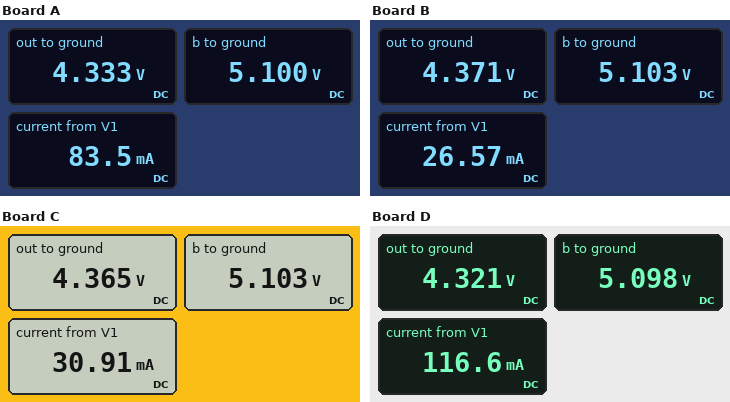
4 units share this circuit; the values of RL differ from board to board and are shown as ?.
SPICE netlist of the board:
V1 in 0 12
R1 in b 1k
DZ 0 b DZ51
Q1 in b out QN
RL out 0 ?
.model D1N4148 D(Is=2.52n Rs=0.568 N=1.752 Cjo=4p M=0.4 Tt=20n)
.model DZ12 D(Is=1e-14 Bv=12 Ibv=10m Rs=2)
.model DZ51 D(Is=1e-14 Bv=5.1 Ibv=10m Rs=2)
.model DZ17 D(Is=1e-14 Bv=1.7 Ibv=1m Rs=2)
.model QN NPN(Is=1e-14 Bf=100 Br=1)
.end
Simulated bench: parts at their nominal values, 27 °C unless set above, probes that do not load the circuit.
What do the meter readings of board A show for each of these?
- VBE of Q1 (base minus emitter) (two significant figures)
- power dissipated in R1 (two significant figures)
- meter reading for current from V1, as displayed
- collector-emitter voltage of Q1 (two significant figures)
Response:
770 mV
48 mW
83.5 mA
7.7 V
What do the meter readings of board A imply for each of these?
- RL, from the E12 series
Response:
56 Ω
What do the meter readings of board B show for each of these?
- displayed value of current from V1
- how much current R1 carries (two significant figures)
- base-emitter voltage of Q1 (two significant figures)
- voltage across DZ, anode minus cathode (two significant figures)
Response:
26.57 mA
6.9 mA
730 mV
-5.1 V
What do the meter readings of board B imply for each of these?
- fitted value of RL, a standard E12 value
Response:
220 Ω
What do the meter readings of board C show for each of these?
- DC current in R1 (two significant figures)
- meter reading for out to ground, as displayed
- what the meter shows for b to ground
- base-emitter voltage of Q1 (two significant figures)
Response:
6.9 mA
4.365 V
5.103 V
740 mV
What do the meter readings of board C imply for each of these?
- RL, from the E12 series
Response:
180 Ω
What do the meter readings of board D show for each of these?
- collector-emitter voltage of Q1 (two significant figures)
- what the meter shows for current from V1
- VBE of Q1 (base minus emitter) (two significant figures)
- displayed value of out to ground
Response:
7.7 V
116.6 mA
780 mV
4.321 V
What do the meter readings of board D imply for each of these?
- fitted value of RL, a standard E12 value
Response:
39 Ω
